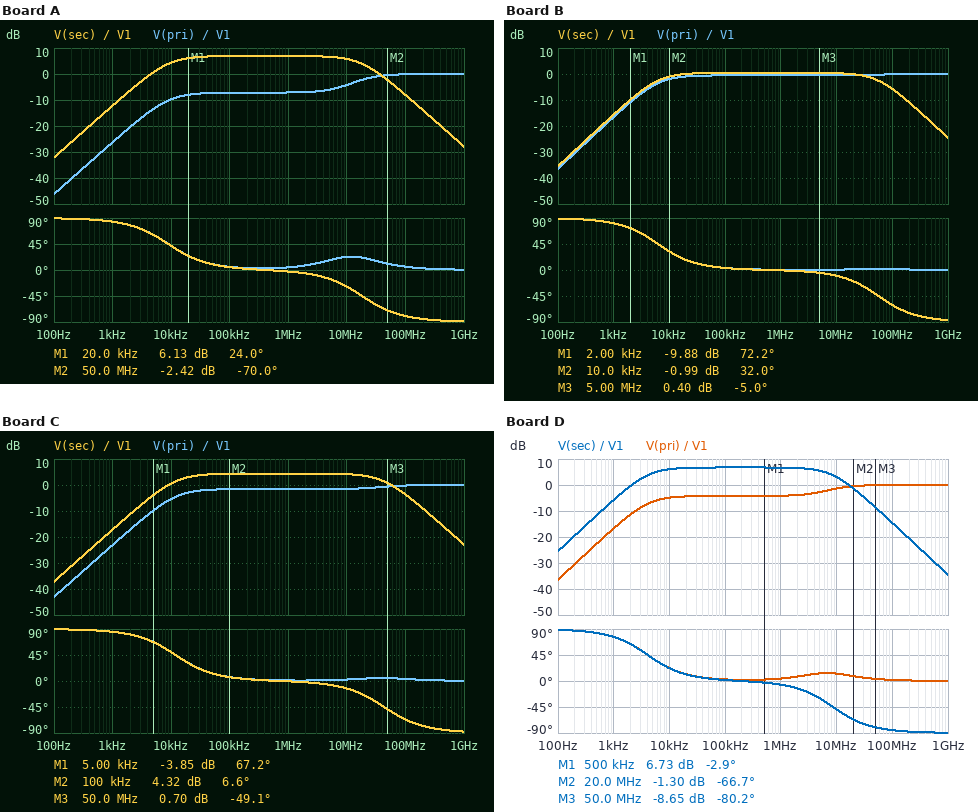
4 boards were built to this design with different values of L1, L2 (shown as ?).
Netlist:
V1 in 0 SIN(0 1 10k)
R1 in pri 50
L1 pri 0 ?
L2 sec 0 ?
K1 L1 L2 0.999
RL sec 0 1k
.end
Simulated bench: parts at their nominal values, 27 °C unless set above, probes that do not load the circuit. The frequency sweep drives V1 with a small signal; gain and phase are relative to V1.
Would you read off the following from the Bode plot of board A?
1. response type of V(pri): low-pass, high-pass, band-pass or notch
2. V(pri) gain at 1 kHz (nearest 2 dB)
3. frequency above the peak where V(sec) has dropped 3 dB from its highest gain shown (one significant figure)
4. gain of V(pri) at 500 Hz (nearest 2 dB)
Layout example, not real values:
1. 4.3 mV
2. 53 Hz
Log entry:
1. high-pass
2. -26 dB
3. 20 MHz
4. -32 dB
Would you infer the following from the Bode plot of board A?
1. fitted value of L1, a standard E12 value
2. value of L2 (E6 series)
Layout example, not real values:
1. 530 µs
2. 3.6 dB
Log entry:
1. 390 µH
2. 10 mH
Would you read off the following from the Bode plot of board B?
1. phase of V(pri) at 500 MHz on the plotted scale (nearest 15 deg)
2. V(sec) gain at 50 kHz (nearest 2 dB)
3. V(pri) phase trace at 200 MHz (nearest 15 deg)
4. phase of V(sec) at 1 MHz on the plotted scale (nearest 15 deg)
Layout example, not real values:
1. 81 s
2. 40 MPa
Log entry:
1. 0 deg
2. 0 dB
3. 0 deg
4. 0 deg
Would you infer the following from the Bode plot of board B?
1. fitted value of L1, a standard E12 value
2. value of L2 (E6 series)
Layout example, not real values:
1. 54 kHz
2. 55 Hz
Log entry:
1. 1.2 mH
2. 1.5 mH
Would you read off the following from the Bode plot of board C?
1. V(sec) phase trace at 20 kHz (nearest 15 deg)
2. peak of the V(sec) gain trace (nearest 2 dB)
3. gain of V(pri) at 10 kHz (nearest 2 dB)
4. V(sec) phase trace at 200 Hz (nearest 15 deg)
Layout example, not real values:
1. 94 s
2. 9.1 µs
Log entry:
1. 30 deg
2. 4 dB
3. -6 dB
4. 90 deg
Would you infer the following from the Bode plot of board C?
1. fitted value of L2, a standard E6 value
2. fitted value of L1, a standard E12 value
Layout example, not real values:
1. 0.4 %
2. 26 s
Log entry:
1. 2.2 mH
2. 560 µH
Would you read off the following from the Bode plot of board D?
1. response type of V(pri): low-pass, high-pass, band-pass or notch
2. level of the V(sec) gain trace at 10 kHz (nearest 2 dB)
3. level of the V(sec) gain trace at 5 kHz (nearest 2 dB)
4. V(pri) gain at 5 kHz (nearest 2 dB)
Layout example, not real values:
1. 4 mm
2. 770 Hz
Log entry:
1. high-pass
2. 6 dB
3. 4 dB
4. -6 dB
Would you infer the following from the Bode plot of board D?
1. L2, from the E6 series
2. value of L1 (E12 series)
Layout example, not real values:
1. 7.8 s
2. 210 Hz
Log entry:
1. 15 mH
2. 1.2 mH
